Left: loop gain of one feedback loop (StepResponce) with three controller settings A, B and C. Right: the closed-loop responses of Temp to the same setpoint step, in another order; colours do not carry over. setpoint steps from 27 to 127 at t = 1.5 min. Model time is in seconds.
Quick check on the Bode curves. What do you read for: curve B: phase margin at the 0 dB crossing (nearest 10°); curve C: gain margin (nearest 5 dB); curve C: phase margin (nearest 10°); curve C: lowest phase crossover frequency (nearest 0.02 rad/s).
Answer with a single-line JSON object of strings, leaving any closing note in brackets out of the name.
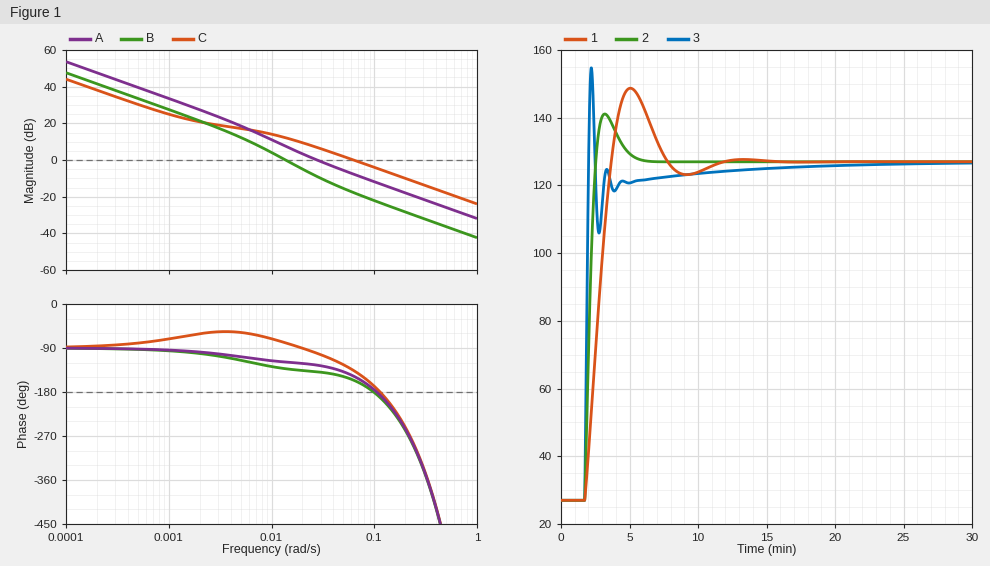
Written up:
{"curve B: phase margin at the 0 dB crossing": "50°", "curve C: gain margin": "5 dB", "curve C: phase margin": "40°", "curve C: lowest phase crossover frequency": "0.12 rad/s"}
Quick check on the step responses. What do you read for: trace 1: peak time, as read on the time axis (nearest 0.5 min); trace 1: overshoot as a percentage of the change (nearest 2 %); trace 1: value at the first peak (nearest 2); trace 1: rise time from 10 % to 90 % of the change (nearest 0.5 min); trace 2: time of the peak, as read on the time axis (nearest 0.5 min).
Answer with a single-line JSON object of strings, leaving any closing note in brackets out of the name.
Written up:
{"trace 1: peak time, as read on the time axis": "5.0 min", "trace 1: overshoot as a percentage of the change": "22 %", "trace 1: value at the first peak": "148", "trace 1: rise time from 10 % to 90 % of the change": "1.5 min", "trace 2: time of the peak, as read on the time axis": "3.0 min"}
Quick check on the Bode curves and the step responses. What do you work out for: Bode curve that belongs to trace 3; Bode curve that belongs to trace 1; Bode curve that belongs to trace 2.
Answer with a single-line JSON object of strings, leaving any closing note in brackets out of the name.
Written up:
{"Bode curve that belongs to trace 3": "C", "Bode curve that belongs to trace 1": "B", "Bode curve that belongs to trace 2": "A"}
